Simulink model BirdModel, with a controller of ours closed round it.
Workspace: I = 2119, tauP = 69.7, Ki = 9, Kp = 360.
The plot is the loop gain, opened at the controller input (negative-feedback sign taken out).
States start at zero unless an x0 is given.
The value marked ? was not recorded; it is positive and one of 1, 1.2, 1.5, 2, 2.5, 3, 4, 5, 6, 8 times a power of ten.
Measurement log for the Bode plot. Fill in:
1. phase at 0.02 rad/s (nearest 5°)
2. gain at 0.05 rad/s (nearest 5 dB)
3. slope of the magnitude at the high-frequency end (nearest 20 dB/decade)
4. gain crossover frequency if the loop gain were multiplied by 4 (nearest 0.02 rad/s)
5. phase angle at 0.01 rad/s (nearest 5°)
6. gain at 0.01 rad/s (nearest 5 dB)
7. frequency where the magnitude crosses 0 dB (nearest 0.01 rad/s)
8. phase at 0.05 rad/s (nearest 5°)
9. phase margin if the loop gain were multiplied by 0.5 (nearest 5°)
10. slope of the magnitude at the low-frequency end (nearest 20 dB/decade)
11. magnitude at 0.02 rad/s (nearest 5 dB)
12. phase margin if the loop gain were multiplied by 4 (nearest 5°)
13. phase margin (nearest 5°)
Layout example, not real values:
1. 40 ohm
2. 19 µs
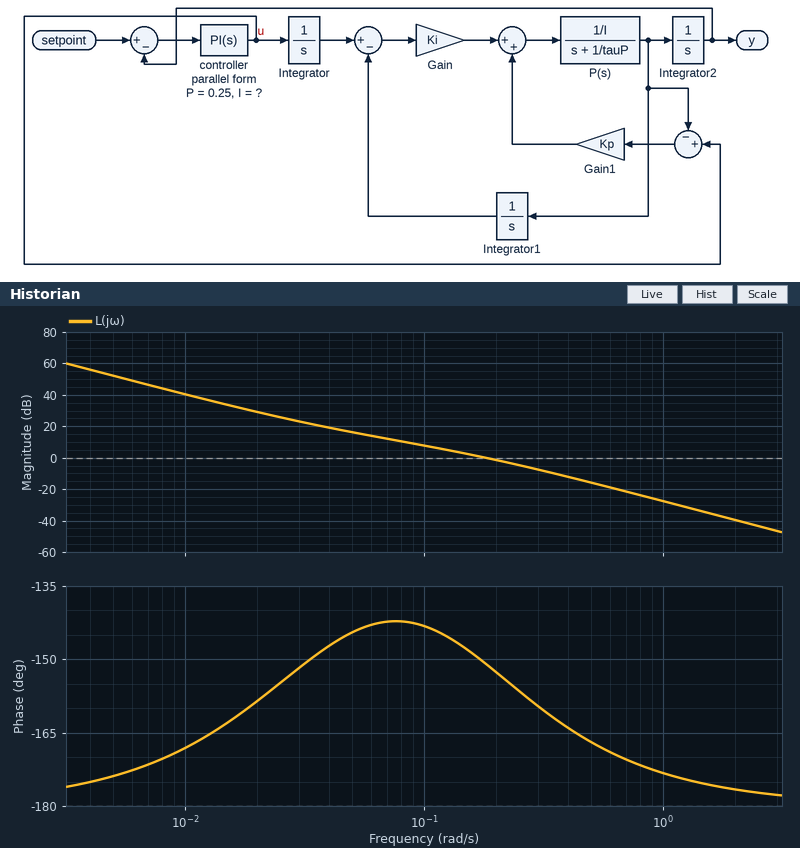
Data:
1. -160°
2. 15 dB
3. -40 dB/decade
4. 0.40 rad/s
5. -170°
6. 40 dB
7. 0.18 rad/s
8. -145°
9. 35°
10. -40 dB/decade
11. 30 dB
12. 15°
13. 30°
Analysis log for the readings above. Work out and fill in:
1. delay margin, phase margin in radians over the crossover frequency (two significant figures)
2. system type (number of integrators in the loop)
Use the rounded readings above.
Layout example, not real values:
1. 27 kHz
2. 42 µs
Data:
1. 2.9 s
2. 2
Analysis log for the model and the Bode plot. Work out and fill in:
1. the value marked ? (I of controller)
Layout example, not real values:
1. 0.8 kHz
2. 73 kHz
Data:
1. 0.01
